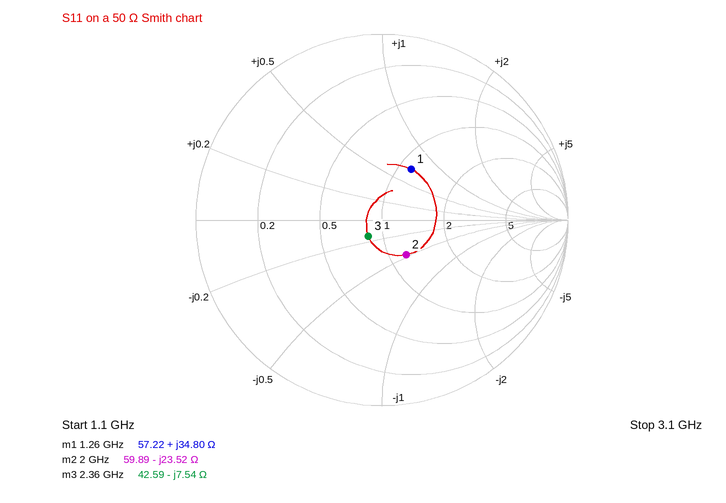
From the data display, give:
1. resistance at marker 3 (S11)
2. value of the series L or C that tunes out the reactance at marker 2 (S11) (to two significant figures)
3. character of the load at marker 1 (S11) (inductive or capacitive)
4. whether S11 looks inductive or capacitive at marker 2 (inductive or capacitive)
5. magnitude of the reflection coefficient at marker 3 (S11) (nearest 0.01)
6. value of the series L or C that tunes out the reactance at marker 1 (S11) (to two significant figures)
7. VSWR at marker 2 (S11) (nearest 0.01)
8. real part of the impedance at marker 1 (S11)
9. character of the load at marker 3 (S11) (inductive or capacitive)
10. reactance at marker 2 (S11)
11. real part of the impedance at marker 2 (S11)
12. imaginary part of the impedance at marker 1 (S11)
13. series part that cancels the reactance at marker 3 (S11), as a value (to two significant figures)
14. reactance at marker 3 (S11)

42.59 Ω
1.9 nH
inductive
capacitive
0.11
3.6 pF
1.59
57.22 Ω
capacitive
-23.52 Ω
59.89 Ω
+34.80 Ω
510 pH
-7.54 Ω
